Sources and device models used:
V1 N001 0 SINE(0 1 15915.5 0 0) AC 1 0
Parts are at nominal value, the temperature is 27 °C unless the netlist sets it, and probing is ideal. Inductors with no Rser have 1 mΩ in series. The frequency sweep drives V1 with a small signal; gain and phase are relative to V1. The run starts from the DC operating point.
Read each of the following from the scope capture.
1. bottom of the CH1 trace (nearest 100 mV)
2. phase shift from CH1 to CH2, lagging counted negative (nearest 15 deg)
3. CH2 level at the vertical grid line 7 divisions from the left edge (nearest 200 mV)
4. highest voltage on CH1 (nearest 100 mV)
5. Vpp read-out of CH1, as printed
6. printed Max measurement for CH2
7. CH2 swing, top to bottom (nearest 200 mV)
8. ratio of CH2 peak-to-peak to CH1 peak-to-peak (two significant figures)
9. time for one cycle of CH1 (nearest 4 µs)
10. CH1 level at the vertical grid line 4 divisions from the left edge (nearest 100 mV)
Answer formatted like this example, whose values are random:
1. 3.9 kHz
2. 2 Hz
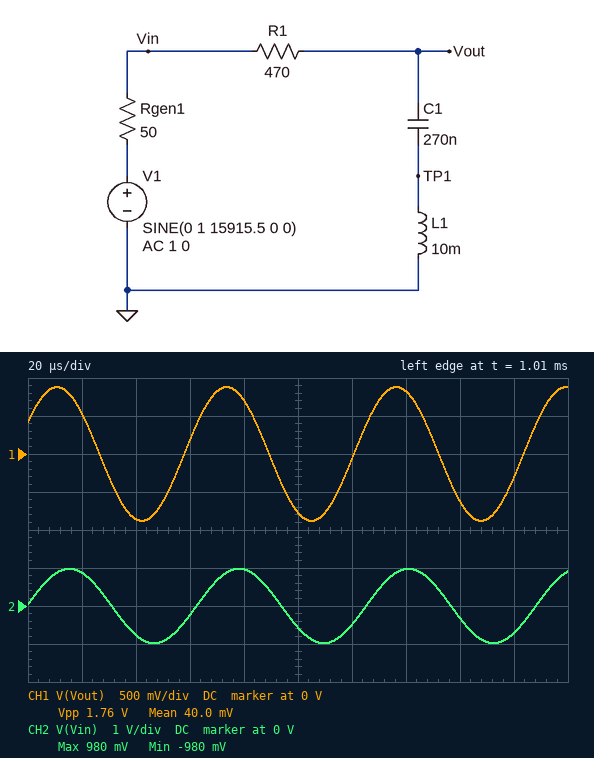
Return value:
1. -900 mV
2. -30 deg
3. 1.0 V
4. 900 mV
5. 1.76 V
6. 980 mV
7. 2.0 V
8. 1.1
9. 64 µs
10. 700 mV
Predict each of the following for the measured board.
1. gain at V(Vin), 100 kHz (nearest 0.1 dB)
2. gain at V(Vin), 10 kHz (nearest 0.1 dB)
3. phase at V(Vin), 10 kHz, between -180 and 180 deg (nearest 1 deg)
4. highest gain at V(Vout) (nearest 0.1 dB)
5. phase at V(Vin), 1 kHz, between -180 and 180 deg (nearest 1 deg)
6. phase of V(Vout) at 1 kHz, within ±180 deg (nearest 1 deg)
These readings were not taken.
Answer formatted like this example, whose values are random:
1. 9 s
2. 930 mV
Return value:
1. 0 dB
2. -0.4 dB
3. 3 deg
4. 0 dB
5. -3 deg
6. -45 deg
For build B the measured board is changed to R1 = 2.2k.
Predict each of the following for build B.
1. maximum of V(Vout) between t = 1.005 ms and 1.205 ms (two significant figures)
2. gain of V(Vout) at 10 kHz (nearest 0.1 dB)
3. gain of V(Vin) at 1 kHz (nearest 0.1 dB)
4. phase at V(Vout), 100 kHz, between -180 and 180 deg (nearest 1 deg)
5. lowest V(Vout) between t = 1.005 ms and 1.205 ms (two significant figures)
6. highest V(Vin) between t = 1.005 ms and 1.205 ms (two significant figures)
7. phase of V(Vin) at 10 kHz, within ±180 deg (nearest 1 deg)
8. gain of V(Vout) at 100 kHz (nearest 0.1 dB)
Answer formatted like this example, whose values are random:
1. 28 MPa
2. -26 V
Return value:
1. 400 mV
2. -12.2 dB
3. -0.2 dB
4. 20 deg
5. -390 mV
6. 980 mV
7. 0 deg
8. -0.5 dB
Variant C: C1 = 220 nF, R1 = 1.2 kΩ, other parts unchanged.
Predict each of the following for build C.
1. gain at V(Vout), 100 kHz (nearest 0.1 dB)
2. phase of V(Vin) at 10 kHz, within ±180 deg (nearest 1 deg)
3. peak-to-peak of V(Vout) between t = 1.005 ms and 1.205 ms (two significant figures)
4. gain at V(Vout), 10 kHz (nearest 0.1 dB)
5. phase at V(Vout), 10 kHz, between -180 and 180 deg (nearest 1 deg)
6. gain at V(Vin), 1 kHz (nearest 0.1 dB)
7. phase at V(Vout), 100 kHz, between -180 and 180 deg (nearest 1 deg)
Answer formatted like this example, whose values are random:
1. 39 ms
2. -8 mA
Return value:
1. -0.2 dB
2. 1 deg
3. 1.2 V
4. -7.8 dB
5. 66 deg
6. -0.3 dB
7. 11 deg
